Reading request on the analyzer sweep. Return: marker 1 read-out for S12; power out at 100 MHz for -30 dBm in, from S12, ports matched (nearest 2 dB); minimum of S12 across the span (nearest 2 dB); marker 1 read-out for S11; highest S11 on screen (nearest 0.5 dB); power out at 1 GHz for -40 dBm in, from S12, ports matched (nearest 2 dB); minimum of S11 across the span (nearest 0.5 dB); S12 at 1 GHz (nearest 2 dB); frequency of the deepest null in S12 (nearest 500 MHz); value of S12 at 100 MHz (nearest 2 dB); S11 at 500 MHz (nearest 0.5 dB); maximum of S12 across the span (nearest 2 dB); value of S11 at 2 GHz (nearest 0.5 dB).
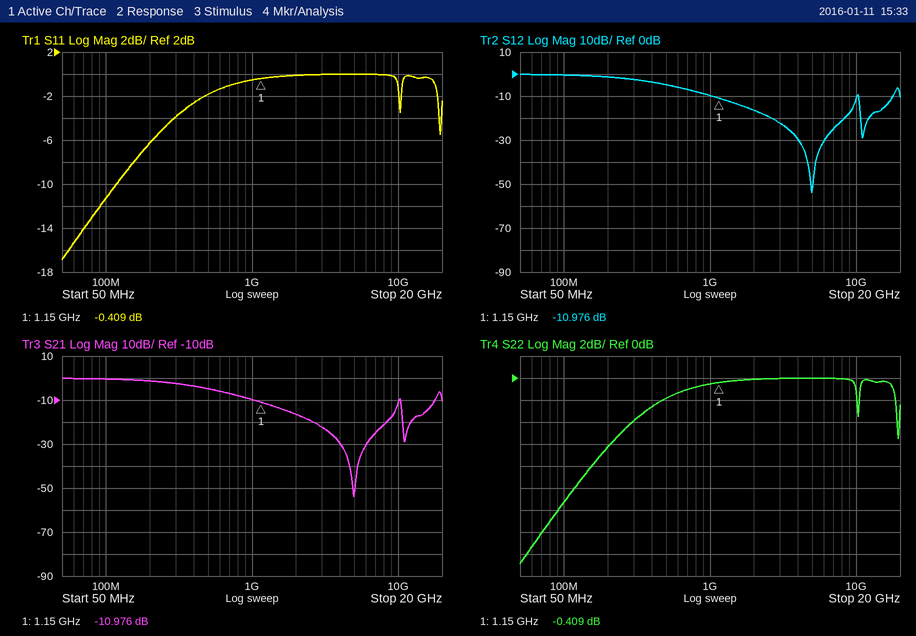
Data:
-10.976 dB
-30 dBm
-54 dB
-0.409 dB
0.0 dB
-50 dBm
-17.0 dB
-10 dB
5.0 GHz
0 dB
-2.0 dB
0 dB
0.0 dB
